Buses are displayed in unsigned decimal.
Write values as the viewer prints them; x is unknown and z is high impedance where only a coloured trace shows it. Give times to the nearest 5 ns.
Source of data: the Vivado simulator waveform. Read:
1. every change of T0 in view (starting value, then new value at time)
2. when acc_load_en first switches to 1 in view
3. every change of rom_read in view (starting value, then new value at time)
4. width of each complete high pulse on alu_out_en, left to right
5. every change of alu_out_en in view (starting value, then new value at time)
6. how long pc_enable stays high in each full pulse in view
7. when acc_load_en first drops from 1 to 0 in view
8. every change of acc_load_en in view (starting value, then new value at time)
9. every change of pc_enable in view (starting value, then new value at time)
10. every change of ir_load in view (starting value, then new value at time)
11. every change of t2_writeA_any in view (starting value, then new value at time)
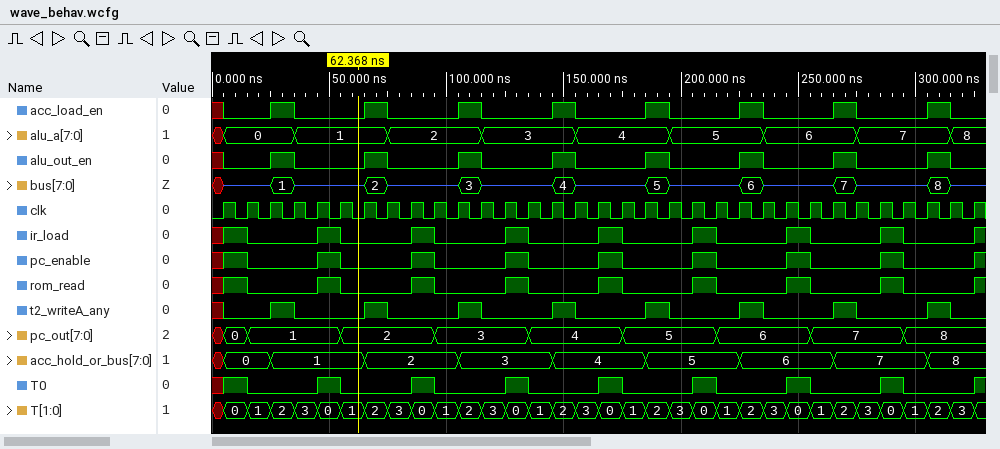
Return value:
x, 1 at 5 ns, 0 at 15 ns, 1 at 45 ns, 0 at 55 ns, 1 at 85 ns, 0 at 95 ns, 1 at 125 ns, 0 at 135 ns, 1 at 165 ns, 0 at 175 ns, 1 at 205 ns, 0 at 215 ns, 1 at 245 ns, 0 at 255 ns, 1 at 285 ns, 0 at 295 ns, 1 at 325 ns
25 ns
x, 1 at 5 ns, 0 at 15 ns, 1 at 45 ns, 0 at 55 ns, 1 at 85 ns, 0 at 95 ns, 1 at 125 ns, 0 at 135 ns, 1 at 165 ns, 0 at 175 ns, 1 at 205 ns, 0 at 215 ns, 1 at 245 ns, 0 at 255 ns, 1 at 285 ns, 0 at 295 ns, 1 at 325 ns
10 ns, 10 ns, 10 ns, 10 ns, 10 ns, 10 ns, 10 ns, 10 ns
x, 0 at 5 ns, 1 at 25 ns, 0 at 35 ns, 1 at 65 ns, 0 at 75 ns, 1 at 105 ns, 0 at 115 ns, 1 at 145 ns, 0 at 155 ns, 1 at 185 ns, 0 at 195 ns, 1 at 225 ns, 0 at 235 ns, 1 at 265 ns, 0 at 275 ns, 1 at 305 ns, 0 at 315 ns
10 ns, 10 ns, 10 ns, 10 ns, 10 ns, 10 ns, 10 ns
35 ns
x, 0 at 5 ns, 1 at 25 ns, 0 at 35 ns, 1 at 65 ns, 0 at 75 ns, 1 at 105 ns, 0 at 115 ns, 1 at 145 ns, 0 at 155 ns, 1 at 185 ns, 0 at 195 ns, 1 at 225 ns, 0 at 235 ns, 1 at 265 ns, 0 at 275 ns, 1 at 305 ns, 0 at 315 ns
x, 1 at 5 ns, 0 at 15 ns, 1 at 45 ns, 0 at 55 ns, 1 at 85 ns, 0 at 95 ns, 1 at 125 ns, 0 at 135 ns, 1 at 165 ns, 0 at 175 ns, 1 at 205 ns, 0 at 215 ns, 1 at 245 ns, 0 at 255 ns, 1 at 285 ns, 0 at 295 ns, 1 at 325 ns
x, 1 at 5 ns, 0 at 15 ns, 1 at 45 ns, 0 at 55 ns, 1 at 85 ns, 0 at 95 ns, 1 at 125 ns, 0 at 135 ns, 1 at 165 ns, 0 at 175 ns, 1 at 205 ns, 0 at 215 ns, 1 at 245 ns, 0 at 255 ns, 1 at 285 ns, 0 at 295 ns, 1 at 325 ns
x, 0 at 5 ns, 1 at 25 ns, 0 at 35 ns, 1 at 65 ns, 0 at 75 ns, 1 at 105 ns, 0 at 115 ns, 1 at 145 ns, 0 at 155 ns, 1 at 185 ns, 0 at 195 ns, 1 at 225 ns, 0 at 235 ns, 1 at 265 ns, 0 at 275 ns, 1 at 305 ns, 0 at 315 ns
